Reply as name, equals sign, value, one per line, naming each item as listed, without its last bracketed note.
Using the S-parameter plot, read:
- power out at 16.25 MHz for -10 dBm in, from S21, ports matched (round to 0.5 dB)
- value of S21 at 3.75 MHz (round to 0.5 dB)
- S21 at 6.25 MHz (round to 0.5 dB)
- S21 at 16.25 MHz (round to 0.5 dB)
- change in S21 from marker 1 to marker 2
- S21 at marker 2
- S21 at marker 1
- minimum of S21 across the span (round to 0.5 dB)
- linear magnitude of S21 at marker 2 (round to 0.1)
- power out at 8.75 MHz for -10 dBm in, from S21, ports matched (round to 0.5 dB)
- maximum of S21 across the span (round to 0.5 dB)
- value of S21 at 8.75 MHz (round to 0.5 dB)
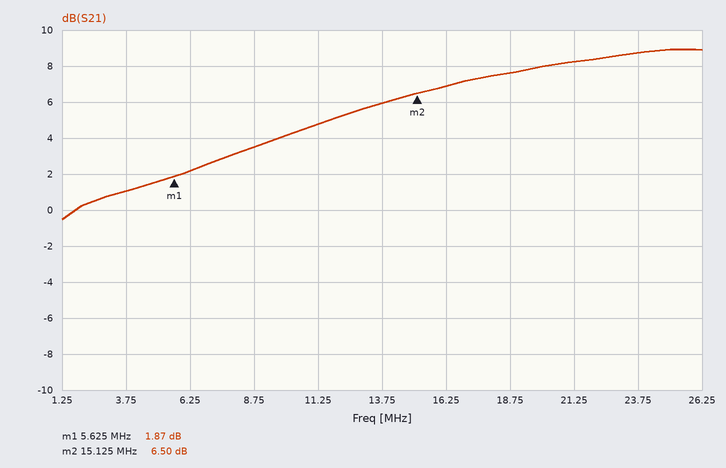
power out at 16.25 MHz for -10 dBm in, from S21, ports matched = -3.0 dBm
value of S21 at 3.75 MHz = 1.0 dB
S21 at 6.25 MHz = 2.0 dB
S21 at 16.25 MHz = 7.0 dB
change in S21 from marker 1 to marker 2 = 4.63 dB
S21 at marker 2 = 6.50 dB
S21 at marker 1 = 1.87 dB
minimum of S21 across the span = -0.5 dB
linear magnitude of S21 at marker 2 = 2.1
power out at 8.75 MHz for -10 dBm in, from S21, ports matched = -6.5 dBm
maximum of S21 across the span = 9.0 dB
value of S21 at 8.75 MHz = 3.5 dB
